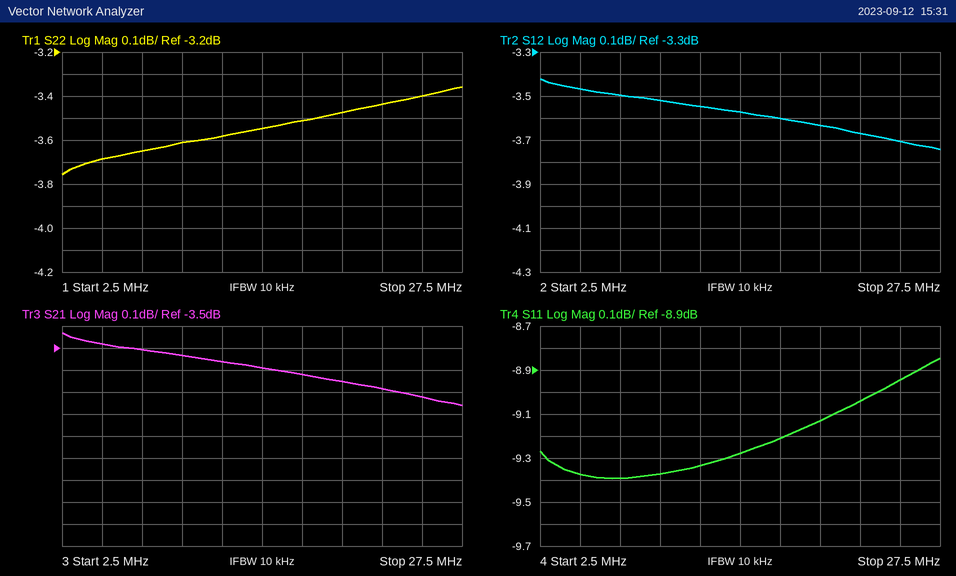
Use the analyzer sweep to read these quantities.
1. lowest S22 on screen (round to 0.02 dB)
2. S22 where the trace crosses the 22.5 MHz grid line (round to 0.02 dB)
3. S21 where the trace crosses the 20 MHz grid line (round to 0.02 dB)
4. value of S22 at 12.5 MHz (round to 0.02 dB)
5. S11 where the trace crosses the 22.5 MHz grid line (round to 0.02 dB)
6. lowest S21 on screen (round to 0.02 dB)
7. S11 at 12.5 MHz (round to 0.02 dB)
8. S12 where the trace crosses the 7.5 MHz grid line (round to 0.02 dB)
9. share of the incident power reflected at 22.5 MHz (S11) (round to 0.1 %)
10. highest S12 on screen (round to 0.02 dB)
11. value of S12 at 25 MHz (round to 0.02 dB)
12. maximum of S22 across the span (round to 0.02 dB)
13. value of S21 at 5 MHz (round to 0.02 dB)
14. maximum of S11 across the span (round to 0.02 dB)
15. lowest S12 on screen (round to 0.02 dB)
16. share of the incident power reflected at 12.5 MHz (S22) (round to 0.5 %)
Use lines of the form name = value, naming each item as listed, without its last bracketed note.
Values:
lowest S22 on screen = -3.76 dB
S22 where the trace crosses the 22.5 MHz grid line = -3.44 dB
S21 where the trace crosses the 20 MHz grid line = -3.66 dB
value of S22 at 12.5 MHz = -3.58 dB
S11 where the trace crosses the 22.5 MHz grid line = -9.04 dB
lowest S21 on screen = -3.76 dB
S11 at 12.5 MHz = -9.34 dB
S12 where the trace crosses the 7.5 MHz grid line = -3.50 dB
share of the incident power reflected at 22.5 MHz (S11) = 12.5 %
highest S12 on screen = -3.42 dB
value of S12 at 25 MHz = -3.70 dB
maximum of S22 across the span = -3.36 dB
value of S21 at 5 MHz = -3.48 dB
maximum of S11 across the span = -8.84 dB
lowest S12 on screen = -3.74 dB
share of the incident power reflected at 12.5 MHz (S22) = 44.0 %
